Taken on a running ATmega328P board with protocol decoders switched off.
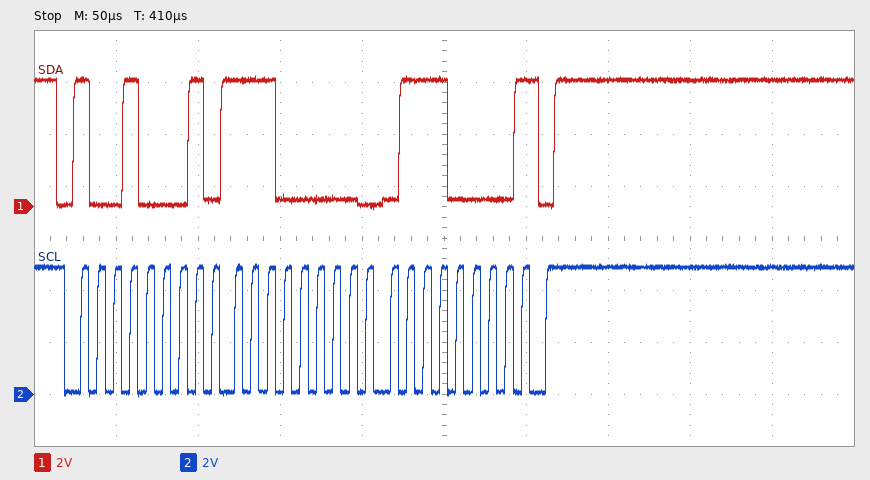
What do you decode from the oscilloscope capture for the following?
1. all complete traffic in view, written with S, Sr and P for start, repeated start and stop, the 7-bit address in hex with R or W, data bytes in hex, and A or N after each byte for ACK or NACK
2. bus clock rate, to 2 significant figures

S 48R A E0 A 70 N P
100 kHz
